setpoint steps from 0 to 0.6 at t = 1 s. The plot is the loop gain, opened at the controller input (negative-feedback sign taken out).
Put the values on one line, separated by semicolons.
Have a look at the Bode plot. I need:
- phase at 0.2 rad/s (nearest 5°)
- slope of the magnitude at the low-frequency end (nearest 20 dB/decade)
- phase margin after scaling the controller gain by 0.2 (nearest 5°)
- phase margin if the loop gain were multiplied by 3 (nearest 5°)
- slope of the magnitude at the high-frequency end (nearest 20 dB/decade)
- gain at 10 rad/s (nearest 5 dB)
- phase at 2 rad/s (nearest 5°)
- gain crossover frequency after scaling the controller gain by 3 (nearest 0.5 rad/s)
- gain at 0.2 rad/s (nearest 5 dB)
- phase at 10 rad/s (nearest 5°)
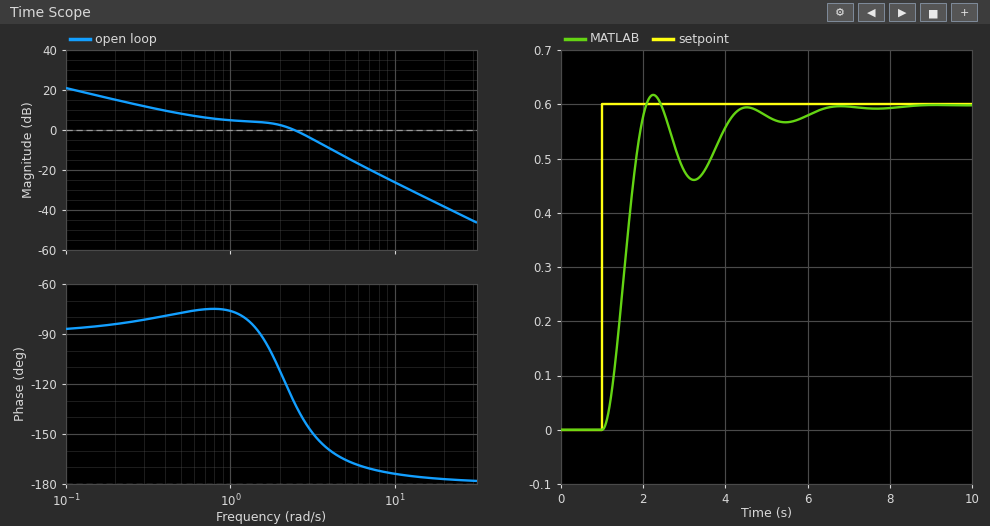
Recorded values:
-85°; -20 dB/decade; 95°; 20°; -40 dB/decade; -25 dB; -110°; 4.0 rad/s; 15 dB; -175°
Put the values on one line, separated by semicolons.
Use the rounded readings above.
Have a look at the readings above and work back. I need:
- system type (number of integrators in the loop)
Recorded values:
1
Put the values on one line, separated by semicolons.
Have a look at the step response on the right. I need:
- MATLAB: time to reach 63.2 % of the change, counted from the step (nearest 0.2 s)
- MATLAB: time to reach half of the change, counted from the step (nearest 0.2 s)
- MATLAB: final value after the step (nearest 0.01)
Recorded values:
0.6 s; 0.6 s; 0.60
